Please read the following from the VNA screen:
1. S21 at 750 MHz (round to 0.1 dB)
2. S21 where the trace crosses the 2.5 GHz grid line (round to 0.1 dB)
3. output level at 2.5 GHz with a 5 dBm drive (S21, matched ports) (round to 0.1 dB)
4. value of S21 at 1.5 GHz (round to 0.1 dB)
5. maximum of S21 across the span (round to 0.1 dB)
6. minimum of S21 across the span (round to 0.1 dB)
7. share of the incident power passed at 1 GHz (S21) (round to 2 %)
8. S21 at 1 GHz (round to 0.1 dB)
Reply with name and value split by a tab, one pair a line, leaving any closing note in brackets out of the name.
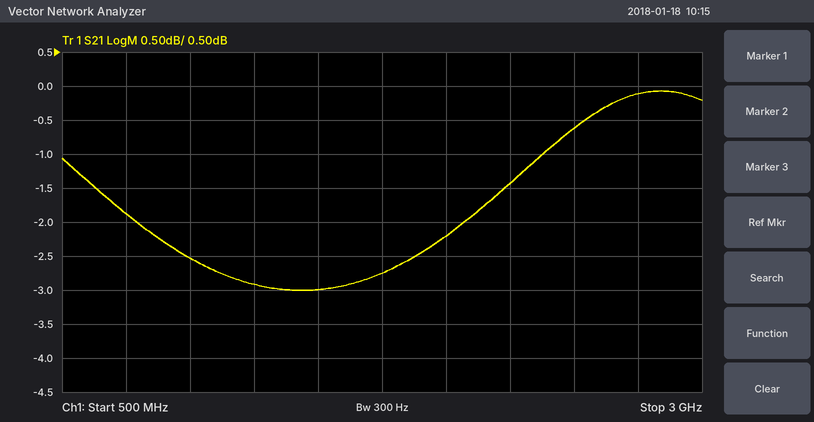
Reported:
S21 at 750 MHz	-1.9 dB
S21 where the trace crosses the 2.5 GHz grid line	-0.6 dB
output level at 2.5 GHz with a 5 dBm drive (S21, matched ports)	4.4 dBm
value of S21 at 1.5 GHz	-3.0 dB
maximum of S21 across the span	-0.1 dB
minimum of S21 across the span	-3.0 dB
share of the incident power passed at 1 GHz (S21)	56 %
S21 at 1 GHz	-2.5 dB
